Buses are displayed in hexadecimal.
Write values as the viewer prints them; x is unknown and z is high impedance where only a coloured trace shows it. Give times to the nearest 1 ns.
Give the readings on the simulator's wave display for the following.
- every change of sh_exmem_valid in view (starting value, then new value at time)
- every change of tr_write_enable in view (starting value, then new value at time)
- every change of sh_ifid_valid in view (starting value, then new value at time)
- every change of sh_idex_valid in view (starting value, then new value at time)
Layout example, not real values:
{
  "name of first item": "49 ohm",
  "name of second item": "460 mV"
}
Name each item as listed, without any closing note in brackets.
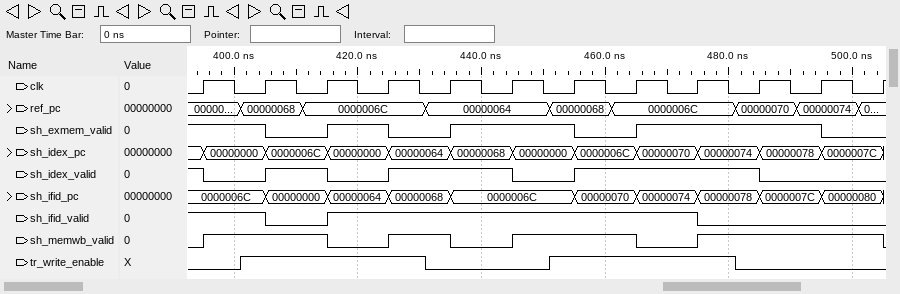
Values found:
{
  "every change of sh_exmem_valid in view": "1, 0 at 405 ns, 1 at 415 ns, 0 at 425 ns, 1 at 435 ns, 0 at 455 ns, 1 at 465 ns, 0 at 495 ns",
  "every change of tr_write_enable in view": "0, 1 at 401 ns, 0 at 431 ns, 1 at 451 ns, 0 at 481 ns",
  "every change of sh_ifid_valid in view": "1, 0 at 405 ns, 1 at 415 ns, 0 at 475 ns",
  "every change of sh_idex_valid in view": "1, 0 at 395 ns, 1 at 405 ns, 0 at 415 ns, 1 at 425 ns, 0 at 445 ns, 1 at 455 ns, 0 at 485 ns"
}
